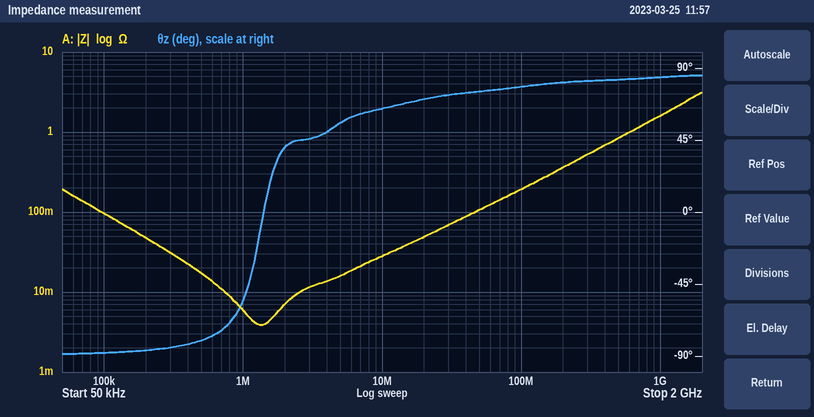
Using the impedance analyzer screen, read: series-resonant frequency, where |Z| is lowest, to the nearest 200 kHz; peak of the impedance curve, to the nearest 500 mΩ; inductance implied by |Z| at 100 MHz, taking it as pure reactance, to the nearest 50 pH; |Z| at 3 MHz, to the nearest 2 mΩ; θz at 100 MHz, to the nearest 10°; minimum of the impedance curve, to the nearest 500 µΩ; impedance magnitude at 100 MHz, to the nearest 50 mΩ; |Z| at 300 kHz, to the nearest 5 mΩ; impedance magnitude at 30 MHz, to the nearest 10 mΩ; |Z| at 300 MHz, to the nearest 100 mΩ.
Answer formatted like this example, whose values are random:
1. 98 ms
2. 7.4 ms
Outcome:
1. 1.4 MHz
2. 3.0 Ω
3. 300 pH
4. 12 mΩ
5. 80°
6. 4.0 mΩ
7. 200 mΩ
8. 30 mΩ
9. 70 mΩ
10. 500 mΩ
